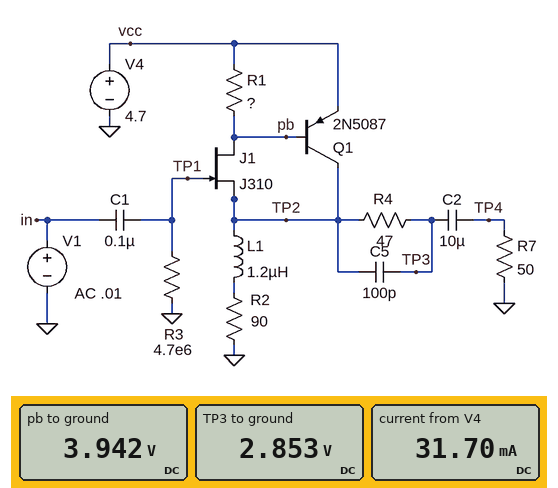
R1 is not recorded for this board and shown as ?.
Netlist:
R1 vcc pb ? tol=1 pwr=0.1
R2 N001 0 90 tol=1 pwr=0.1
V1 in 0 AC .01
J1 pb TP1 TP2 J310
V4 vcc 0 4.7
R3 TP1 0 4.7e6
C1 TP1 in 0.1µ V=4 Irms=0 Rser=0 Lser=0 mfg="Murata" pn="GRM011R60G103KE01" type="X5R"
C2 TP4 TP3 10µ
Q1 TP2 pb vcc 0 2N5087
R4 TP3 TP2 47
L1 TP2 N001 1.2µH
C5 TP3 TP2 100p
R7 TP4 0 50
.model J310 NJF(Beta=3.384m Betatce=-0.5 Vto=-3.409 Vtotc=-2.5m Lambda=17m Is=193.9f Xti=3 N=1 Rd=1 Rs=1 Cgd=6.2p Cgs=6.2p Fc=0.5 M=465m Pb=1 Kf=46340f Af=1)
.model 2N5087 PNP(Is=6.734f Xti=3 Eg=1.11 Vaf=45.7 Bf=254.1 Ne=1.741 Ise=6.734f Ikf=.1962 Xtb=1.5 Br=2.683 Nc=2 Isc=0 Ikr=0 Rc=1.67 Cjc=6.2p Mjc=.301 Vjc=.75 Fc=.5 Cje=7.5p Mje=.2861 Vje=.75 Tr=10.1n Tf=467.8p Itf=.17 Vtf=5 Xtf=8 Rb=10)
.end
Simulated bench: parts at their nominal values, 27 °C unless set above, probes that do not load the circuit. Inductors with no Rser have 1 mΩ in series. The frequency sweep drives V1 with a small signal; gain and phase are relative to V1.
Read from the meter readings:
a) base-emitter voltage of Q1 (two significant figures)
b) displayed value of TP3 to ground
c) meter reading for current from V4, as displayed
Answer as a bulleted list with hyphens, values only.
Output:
- -760 mV
- 2.853 V
- 31.70 mA
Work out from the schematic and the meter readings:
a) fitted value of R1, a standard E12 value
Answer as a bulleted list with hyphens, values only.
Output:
- 820 Ω
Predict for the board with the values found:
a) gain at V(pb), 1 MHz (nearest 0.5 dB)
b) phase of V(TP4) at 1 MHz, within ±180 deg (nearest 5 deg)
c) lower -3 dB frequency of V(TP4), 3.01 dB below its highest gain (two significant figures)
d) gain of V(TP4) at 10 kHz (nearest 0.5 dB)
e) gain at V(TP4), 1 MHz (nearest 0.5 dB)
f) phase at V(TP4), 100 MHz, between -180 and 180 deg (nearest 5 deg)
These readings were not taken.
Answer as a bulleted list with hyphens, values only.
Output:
- -33.5 dB
- 0 deg
- 160 Hz
- -6.0 dB
- -6.0 dB
- -75 deg
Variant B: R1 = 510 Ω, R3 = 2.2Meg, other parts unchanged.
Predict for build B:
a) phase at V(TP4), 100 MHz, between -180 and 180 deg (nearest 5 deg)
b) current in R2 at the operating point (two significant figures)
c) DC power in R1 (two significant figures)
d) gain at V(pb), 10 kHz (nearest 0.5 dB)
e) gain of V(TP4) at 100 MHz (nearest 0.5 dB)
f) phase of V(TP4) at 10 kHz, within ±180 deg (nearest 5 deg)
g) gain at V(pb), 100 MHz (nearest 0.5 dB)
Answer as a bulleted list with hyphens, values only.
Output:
- -65 deg
- 30 mA
- 1.1 mW
- -33.0 dB
- -12.0 dB
- 0 deg
- -27.0 dB
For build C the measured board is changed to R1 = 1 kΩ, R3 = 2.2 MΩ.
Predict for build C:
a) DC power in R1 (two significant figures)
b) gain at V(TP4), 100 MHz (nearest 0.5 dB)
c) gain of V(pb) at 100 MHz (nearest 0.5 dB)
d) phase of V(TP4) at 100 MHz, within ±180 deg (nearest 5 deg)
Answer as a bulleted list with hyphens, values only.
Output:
- 580 µW
- -15.5 dB
- -28.5 dB
- -80 deg
